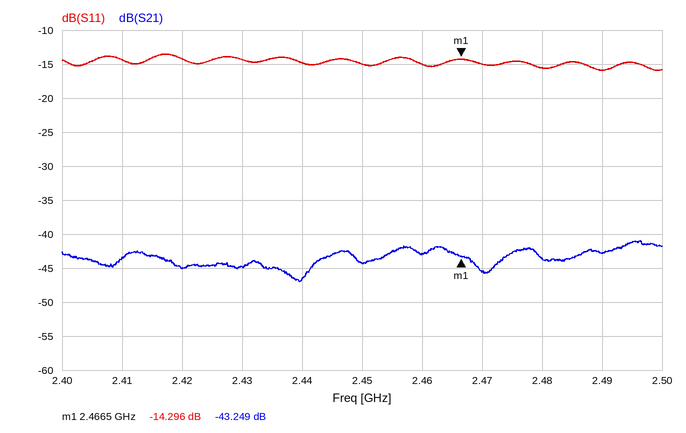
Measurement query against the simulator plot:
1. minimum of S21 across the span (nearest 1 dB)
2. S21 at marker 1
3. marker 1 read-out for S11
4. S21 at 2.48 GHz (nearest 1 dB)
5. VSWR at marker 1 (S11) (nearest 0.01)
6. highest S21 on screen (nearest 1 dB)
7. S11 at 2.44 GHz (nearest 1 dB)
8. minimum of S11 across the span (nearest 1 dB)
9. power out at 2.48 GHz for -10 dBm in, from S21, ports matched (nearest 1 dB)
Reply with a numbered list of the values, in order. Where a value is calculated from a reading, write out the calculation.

1. -47 dB
2. -43.249 dB
3. -14.296 dB
4. -44 dB
5. (1 + 0.1928)/(1 − 0.1928) ≈ 1.48
6. -41 dB
7. -15 dB
8. -16 dB
9. -10 dBm + (-44 dB) = -54 dBm
